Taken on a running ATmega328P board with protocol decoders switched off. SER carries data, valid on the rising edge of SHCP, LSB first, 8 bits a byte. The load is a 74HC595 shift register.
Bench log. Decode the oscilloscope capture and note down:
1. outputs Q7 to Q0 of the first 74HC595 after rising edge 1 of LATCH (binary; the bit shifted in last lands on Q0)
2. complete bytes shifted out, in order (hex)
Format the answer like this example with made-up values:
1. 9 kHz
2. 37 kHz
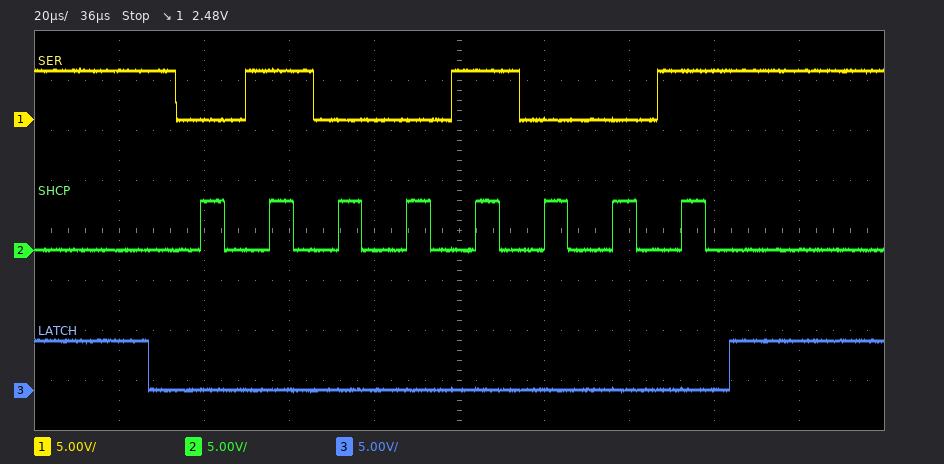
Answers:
1. 01001001
2. 92
